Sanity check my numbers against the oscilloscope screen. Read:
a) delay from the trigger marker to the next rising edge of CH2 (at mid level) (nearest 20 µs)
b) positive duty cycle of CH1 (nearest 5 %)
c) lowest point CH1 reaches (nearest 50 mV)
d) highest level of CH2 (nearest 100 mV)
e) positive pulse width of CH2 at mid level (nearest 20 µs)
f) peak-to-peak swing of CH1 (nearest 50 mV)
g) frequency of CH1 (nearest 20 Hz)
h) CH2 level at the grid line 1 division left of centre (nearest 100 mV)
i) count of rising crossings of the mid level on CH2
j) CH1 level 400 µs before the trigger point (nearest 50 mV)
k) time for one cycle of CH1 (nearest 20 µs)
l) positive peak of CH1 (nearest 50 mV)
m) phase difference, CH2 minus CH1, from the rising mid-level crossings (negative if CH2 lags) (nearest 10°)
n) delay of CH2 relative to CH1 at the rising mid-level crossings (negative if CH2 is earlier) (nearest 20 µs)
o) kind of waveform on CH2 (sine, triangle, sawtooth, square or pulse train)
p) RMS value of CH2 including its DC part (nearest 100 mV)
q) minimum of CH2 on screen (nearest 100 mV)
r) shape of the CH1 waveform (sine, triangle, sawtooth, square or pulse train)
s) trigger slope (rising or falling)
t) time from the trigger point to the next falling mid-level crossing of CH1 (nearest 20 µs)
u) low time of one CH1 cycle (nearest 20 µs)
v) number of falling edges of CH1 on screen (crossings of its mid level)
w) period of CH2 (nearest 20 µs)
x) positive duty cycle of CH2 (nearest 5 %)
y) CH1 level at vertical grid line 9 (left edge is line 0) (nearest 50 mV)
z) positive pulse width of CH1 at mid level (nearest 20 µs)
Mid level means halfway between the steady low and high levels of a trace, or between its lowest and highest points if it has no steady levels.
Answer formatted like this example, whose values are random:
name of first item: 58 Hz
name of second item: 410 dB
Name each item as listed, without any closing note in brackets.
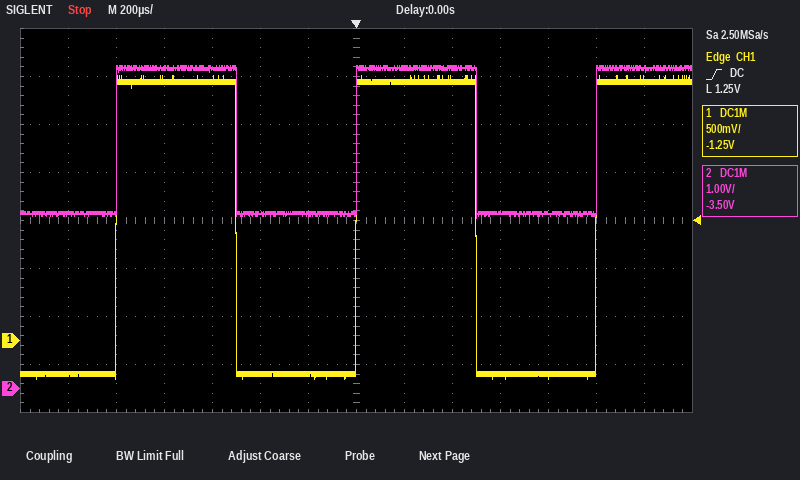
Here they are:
delay from the trigger marker to the next rising edge of CH2 (at mid level): 1.00 ms
positive duty cycle of CH1: 50 %
lowest point CH1 reaches: -400 mV
highest level of CH2: 6.7 V
positive pulse width of CH2 at mid level: 500 µs
peak-to-peak swing of CH1: 3.15 V
frequency of CH1: 1.00 kHz
CH2 level at the grid line 1 division left of centre: 3.6 V
count of rising crossings of the mid level on CH2: 3
CH1 level 400 µs before the trigger point: -350 mV
time for one cycle of CH1: 1.00 ms
positive peak of CH1: 2.75 V
phase difference, CH2 minus CH1, from the rising mid-level crossings (negative if CH2 lags): 0°
delay of CH2 relative to CH1 at the rising mid-level crossings (negative if CH2 is earlier): 0 µs
kind of waveform on CH2: square
RMS value of CH2 including its DC part: 5.4 V
minimum of CH2 on screen: 3.6 V
shape of the CH1 waveform: square
trigger slope: rising
time from the trigger point to the next falling mid-level crossing of CH1: 500 µs
low time of one CH1 cycle: 500 µs
number of falling edges of CH1 on screen: 2
period of CH2: 1.00 ms
positive duty cycle of CH2: 50 %
CH1 level at vertical grid line 9 (left edge is line 0): 2.70 V
positive pulse width of CH1 at mid level: 500 µs
